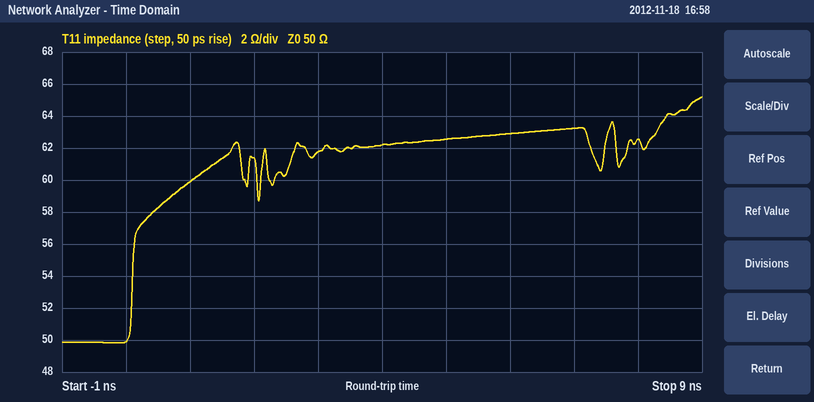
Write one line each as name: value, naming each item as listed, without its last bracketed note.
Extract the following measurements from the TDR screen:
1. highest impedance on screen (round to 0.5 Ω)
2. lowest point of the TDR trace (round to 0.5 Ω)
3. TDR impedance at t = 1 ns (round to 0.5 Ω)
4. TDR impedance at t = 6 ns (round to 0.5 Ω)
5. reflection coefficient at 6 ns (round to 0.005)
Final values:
highest impedance on screen: 65.0 Ω
lowest point of the TDR trace: 50.0 Ω
TDR impedance at t = 1 ns: 60.0 Ω
TDR impedance at t = 6 ns: 63.0 Ω
reflection coefficient at 6 ns: +0.115
